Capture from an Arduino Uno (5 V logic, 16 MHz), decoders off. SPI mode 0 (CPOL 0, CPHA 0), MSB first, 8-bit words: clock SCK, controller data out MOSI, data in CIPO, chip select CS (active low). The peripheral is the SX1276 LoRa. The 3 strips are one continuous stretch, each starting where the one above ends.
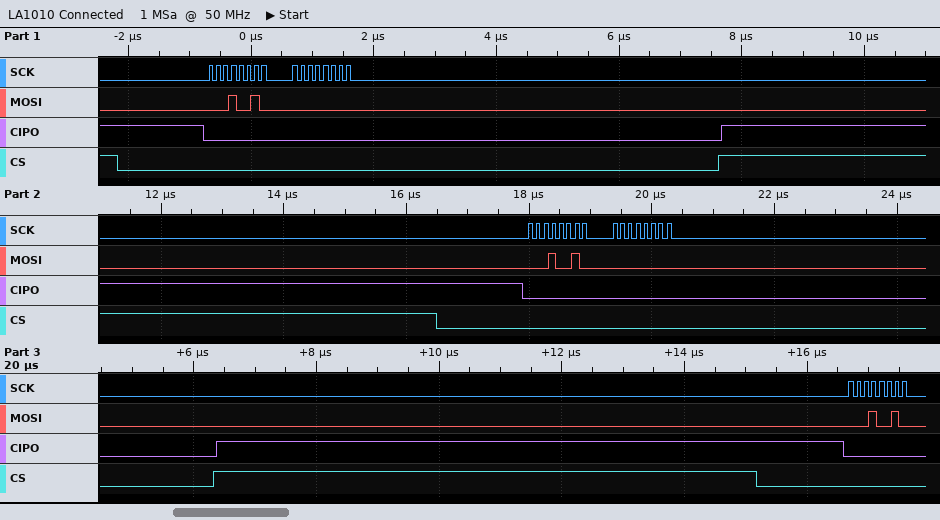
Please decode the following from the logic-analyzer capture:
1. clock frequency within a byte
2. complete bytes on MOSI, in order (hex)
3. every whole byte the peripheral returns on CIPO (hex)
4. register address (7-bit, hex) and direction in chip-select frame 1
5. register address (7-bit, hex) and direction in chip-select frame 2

8 MHz
0x12 0x00 0x12 0x00 0x12
0x00 0x00 0x00 0x00 0x00
0x12 read
0x12 read
